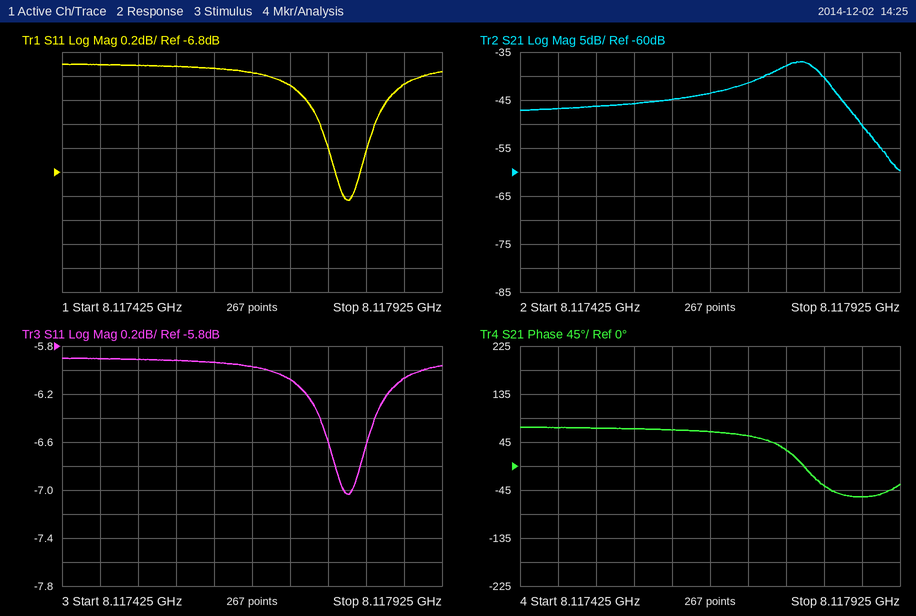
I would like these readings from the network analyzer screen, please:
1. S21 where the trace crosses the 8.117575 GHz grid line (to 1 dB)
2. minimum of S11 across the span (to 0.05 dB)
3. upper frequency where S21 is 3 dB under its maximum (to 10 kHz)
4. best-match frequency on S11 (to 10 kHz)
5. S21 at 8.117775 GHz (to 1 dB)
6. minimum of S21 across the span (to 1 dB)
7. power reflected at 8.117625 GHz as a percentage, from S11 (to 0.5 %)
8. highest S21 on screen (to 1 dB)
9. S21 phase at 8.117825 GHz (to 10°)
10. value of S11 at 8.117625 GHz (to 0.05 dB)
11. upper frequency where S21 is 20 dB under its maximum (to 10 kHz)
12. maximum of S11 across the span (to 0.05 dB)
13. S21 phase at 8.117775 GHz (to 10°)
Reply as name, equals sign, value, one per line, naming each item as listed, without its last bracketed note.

S21 where the trace crosses the 8.117575 GHz grid line = -46 dB
minimum of S11 across the span = -7.05 dB
upper frequency where S21 is 3 dB under its maximum = 8.11782 GHz
best-match frequency on S11 = 8.11780 GHz
S21 at 8.117775 GHz = -38 dB
minimum of S21 across the span = -60 dB
power reflected at 8.117625 GHz as a percentage, from S11 = 25.5 %
highest S21 on screen = -37 dB
S21 phase at 8.117825 GHz = -40°
value of S11 at 8.117625 GHz = -5.95 dB
upper frequency where S21 is 20 dB under its maximum = 8.11791 GHz
maximum of S11 across the span = -5.90 dB
S21 phase at 8.117775 GHz = 30°
